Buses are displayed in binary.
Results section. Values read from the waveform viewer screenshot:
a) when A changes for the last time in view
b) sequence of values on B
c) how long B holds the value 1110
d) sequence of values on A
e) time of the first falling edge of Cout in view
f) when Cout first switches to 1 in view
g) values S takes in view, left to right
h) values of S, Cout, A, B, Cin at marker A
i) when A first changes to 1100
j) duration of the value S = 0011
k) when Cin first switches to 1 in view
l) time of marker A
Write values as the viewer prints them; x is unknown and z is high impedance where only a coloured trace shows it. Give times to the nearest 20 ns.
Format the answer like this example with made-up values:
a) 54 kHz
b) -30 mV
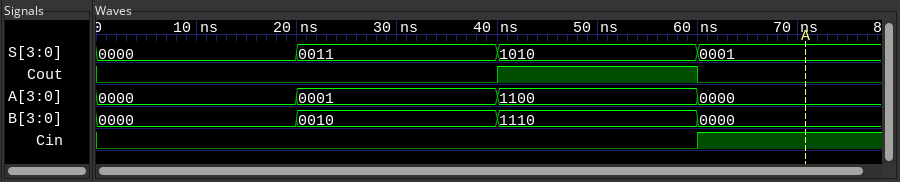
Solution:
a) 60 ns
b) 0000, 0010, 1110, 0000
c) 20 ns
d) 0000, 0001, 1100, 0000
e) 60 ns
f) 40 ns
g) 0000, 0011, 1010, 0001
h) S=0001, Cout=0, A=0000, B=0000, Cin=1
i) 40 ns
j) 20 ns
k) 60 ns
l) 80 ns
